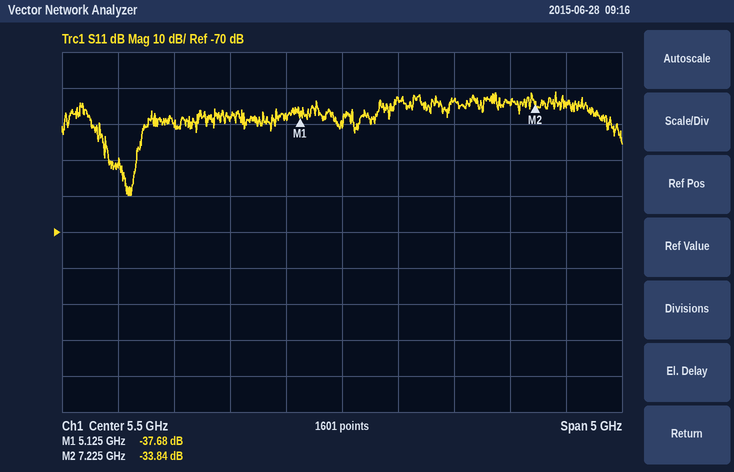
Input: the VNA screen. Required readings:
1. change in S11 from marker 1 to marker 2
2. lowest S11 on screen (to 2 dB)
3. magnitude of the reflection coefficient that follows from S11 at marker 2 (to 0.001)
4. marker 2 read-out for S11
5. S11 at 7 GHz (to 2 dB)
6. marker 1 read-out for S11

3.84 dB
-60 dB
0.020
-33.84 dB
-34 dB
-37.68 dB
